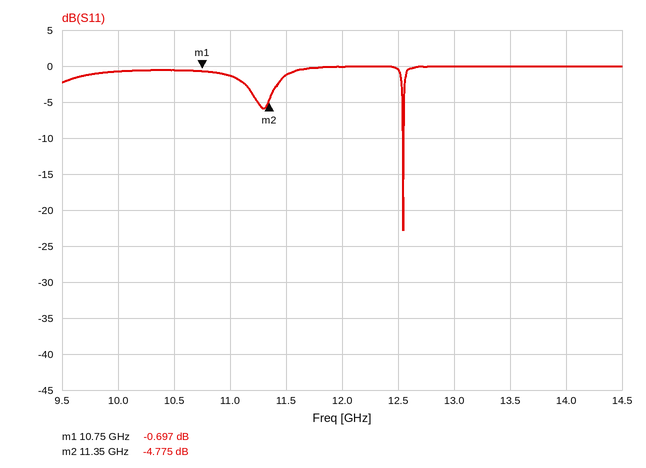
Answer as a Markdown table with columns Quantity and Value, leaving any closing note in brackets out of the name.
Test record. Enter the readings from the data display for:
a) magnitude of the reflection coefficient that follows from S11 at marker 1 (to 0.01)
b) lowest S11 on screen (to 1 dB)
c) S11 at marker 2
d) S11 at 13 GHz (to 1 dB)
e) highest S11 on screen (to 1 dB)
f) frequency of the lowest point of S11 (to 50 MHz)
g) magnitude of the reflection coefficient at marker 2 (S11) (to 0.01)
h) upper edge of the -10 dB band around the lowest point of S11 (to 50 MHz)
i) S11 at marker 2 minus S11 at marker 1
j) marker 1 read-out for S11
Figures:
| Quantity | Value |
|---|---|
| magnitude of the reflection coefficient that follows from S11 at marker 1 | 0.92 |
| lowest S11 on screen | -23 dB |
| S11 at marker 2 | -4.775 dB |
| S11 at 13 GHz | 0 dB |
| highest S11 on screen | 0 dB |
| frequency of the lowest point of S11 | 12.55 GHz |
| magnitude of the reflection coefficient at marker 2 (S11) | 0.58 |
| upper edge of the -10 dB band around the lowest point of S11 | 12.55 GHz |
| S11 at marker 2 minus S11 at marker 1 | -4.078 dB |
| marker 1 read-out for S11 | -0.697 dB |
